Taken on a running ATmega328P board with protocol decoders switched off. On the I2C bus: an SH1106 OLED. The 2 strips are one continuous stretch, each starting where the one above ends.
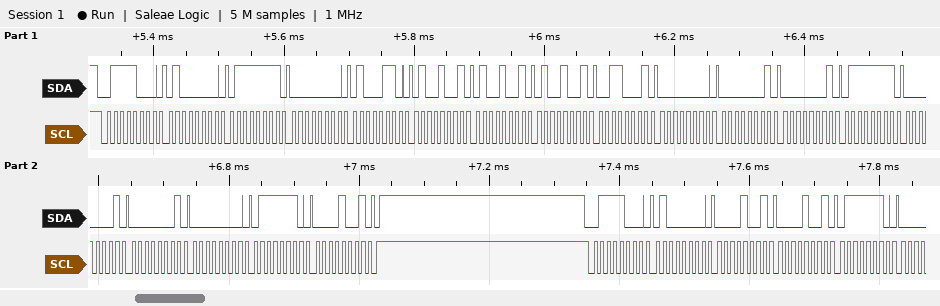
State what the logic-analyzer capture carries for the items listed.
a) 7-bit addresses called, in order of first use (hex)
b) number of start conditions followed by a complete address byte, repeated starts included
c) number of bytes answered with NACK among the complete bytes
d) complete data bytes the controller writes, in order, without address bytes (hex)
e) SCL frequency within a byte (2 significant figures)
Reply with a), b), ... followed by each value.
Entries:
a) 0x3C
b) 2
c) 0
d) 40 7F 00 46 49 49 49 31 00 01 01 7F 01 01 00 7E 09 40 09 09 7E
e) 100 kHz
